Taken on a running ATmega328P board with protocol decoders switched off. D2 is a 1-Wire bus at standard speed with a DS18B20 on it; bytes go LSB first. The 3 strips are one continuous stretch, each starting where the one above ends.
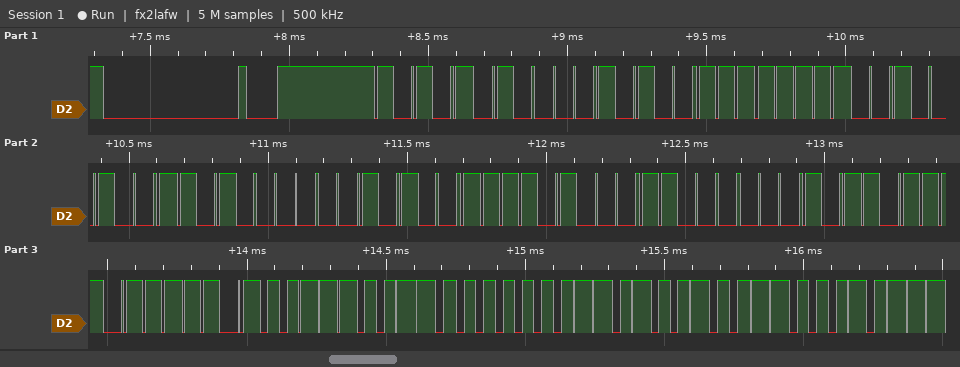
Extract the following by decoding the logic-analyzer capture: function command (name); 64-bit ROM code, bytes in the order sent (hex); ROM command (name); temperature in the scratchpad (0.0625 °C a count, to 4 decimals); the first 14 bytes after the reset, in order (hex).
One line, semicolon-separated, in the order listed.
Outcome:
Read Scratchpad; 28 FF 24 0B 94 17 03 ED; Match ROM; 25.7500 °C; 55 28 FF 24 0B 94 17 03 ED BE 9C 01 4B 46
